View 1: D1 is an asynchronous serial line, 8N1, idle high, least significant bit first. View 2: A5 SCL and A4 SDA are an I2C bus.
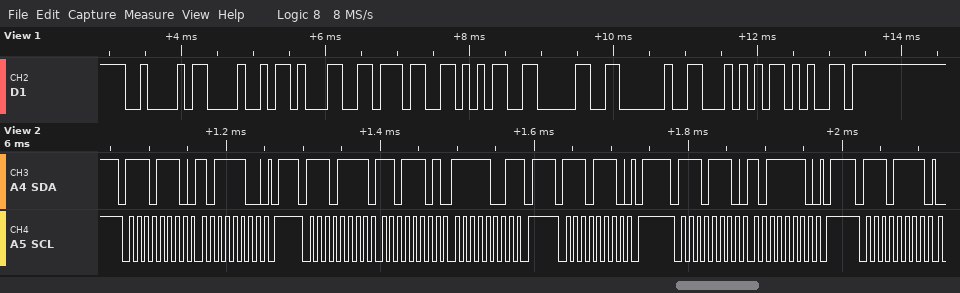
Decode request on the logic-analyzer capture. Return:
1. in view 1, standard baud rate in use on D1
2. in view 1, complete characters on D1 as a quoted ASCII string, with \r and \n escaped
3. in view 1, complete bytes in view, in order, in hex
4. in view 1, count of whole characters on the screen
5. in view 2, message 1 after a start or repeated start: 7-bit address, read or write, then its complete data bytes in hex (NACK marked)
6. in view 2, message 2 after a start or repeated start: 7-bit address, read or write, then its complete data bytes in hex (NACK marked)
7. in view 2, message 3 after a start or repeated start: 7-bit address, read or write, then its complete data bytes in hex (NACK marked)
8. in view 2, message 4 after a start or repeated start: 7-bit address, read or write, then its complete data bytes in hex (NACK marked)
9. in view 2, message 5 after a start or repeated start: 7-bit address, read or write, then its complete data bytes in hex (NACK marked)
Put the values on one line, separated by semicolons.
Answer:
9600 baud; "BH1750 Te"; 42 48 31 37 35 30 20 54 65; 9; 0x77 write: BC; 0x77 read: DD F9 NACK; 0x77 write; 0x77 write: BE; 0x77 read
